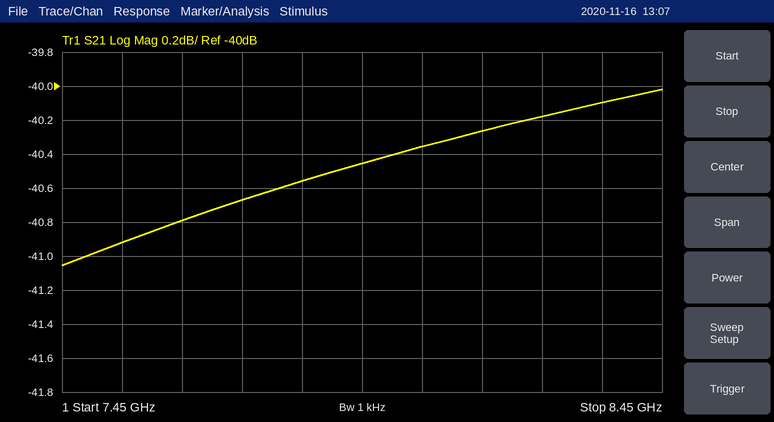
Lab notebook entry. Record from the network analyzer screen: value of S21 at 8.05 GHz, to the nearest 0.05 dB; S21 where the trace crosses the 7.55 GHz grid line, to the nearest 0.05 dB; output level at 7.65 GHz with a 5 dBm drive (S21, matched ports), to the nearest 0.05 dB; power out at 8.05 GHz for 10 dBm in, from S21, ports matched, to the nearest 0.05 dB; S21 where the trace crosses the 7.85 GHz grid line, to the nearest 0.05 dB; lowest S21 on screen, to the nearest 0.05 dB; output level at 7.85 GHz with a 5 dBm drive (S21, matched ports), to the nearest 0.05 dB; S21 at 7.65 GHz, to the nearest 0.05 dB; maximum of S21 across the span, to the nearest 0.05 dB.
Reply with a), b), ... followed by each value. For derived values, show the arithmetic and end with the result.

a) -40.35 dB
b) -40.90 dB
c) 5 dBm + (-40.80 dB) = -35.80 dBm
d) 10 dBm + (-40.35 dB) = -30.35 dBm
e) -40.55 dB
f) -41.05 dB
g) 5 dBm + (-40.55 dB) = -35.55 dBm
h) -40.80 dB
i) -40.00 dB
